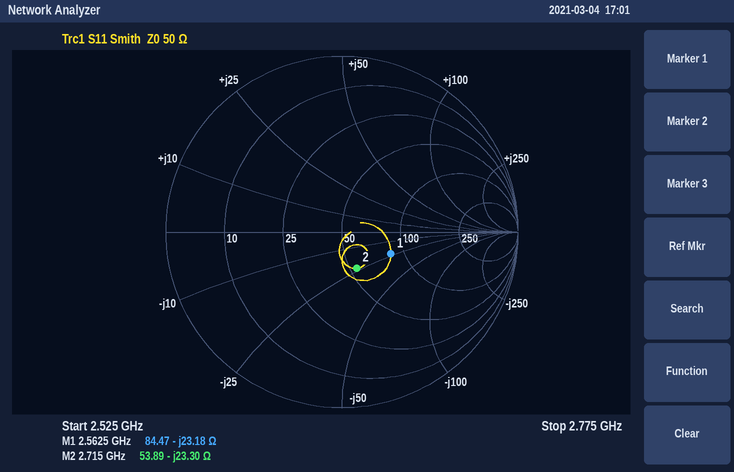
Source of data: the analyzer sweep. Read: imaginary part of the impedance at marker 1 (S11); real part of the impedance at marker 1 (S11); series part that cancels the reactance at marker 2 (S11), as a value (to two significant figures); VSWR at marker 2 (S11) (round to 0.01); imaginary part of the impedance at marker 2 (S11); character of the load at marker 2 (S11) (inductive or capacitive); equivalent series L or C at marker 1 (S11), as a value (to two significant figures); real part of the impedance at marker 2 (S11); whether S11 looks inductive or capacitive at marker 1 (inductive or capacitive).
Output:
-23.18 Ω
84.47 Ω
1.4 nH
1.57
-23.30 Ω
capacitive
2.7 pF
53.89 Ω
capacitive
